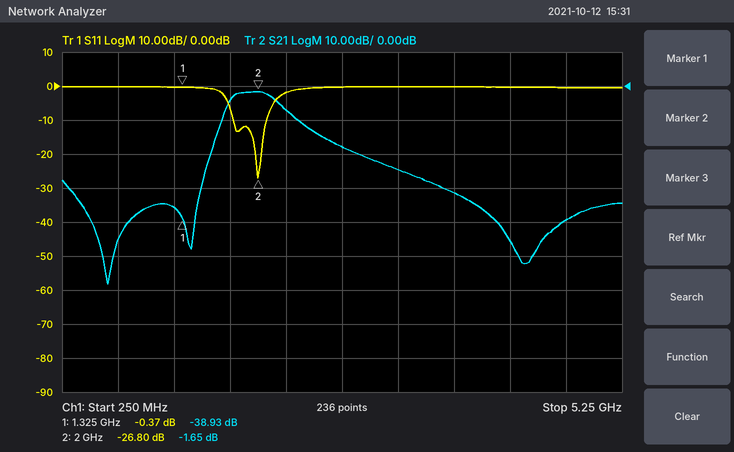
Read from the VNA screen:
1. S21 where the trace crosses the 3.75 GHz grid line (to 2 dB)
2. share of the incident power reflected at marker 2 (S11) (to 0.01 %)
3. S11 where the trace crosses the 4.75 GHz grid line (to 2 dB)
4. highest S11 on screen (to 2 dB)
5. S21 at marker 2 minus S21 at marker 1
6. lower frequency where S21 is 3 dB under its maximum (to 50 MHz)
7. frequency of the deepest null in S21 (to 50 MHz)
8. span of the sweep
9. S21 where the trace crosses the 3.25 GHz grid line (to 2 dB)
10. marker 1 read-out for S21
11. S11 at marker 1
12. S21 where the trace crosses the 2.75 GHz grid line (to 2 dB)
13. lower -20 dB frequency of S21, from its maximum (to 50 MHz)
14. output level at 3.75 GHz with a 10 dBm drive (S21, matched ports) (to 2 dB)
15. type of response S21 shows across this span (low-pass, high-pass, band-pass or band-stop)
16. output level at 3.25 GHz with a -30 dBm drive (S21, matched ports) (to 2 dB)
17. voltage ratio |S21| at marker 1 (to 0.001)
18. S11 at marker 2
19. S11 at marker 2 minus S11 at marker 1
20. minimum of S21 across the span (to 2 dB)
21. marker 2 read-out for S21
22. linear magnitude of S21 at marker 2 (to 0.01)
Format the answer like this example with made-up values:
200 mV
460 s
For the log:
-32 dB
0.21 %
0 dB
0 dB
37.28 dB
1.75 GHz
650 MHz
5 GHz
-24 dB
-38.93 dB
-0.37 dB
-18 dB
1.55 GHz
-22 dBm
band-pass
-54 dBm
0.011
-26.80 dB
-26.43 dB
-58 dB
-1.65 dB
0.83
